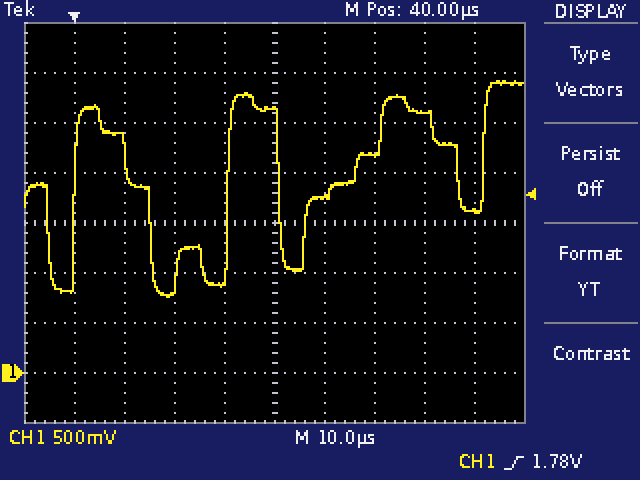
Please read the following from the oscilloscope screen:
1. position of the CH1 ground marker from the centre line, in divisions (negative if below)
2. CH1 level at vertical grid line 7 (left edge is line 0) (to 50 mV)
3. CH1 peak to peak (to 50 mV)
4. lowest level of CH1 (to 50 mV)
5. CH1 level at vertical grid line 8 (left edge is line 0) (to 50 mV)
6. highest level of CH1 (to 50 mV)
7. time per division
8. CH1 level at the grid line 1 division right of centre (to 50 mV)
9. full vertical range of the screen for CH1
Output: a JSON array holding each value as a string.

["-3.0 div", "2.20 V", "2.15 V", "750 mV", "2.60 V", "2.90 V", "10 µs", "1.75 V", "4 V"]
